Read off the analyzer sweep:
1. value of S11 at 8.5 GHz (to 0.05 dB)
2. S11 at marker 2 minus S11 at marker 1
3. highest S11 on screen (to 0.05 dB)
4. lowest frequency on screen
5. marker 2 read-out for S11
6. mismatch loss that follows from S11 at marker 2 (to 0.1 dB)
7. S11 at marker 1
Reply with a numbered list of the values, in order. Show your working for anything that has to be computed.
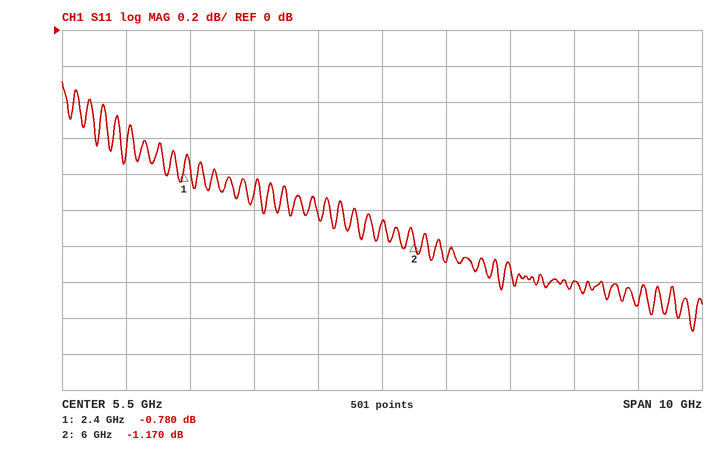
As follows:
1. -1.40 dB
2. -1.17 − (-0.78) = -0.390 dB
3. -0.30 dB
4. 500 MHz
5. -1.170 dB
6. −10 log10(1 − 10^(-1.17/10)) ≈ 6.3 dB
7. -0.780 dB
